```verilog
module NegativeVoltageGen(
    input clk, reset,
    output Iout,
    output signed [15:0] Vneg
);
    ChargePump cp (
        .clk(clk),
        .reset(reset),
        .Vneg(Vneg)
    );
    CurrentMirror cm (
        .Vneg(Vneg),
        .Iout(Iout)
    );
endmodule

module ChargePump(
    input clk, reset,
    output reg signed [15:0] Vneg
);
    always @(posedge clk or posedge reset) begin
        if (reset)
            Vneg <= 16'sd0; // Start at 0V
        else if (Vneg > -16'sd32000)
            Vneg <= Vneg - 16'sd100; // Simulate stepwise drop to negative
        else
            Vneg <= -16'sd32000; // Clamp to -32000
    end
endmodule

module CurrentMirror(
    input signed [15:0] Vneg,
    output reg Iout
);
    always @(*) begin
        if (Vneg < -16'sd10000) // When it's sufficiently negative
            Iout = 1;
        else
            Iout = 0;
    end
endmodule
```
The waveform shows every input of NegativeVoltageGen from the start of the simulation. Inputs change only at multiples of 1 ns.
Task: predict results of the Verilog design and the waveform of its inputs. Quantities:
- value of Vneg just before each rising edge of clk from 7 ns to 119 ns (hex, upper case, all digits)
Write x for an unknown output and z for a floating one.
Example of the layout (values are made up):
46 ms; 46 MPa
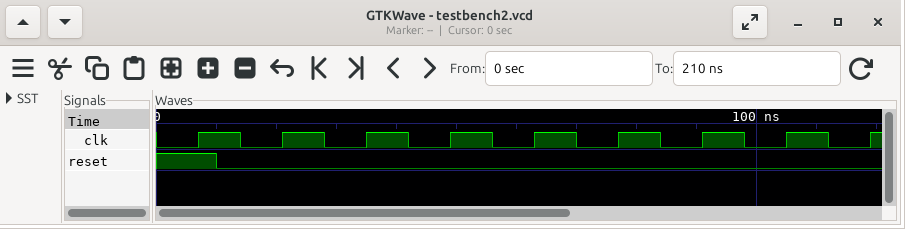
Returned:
0000, 0000, FF9C, FF38, FED4, FE70, FE0C, FDA8, FD44
